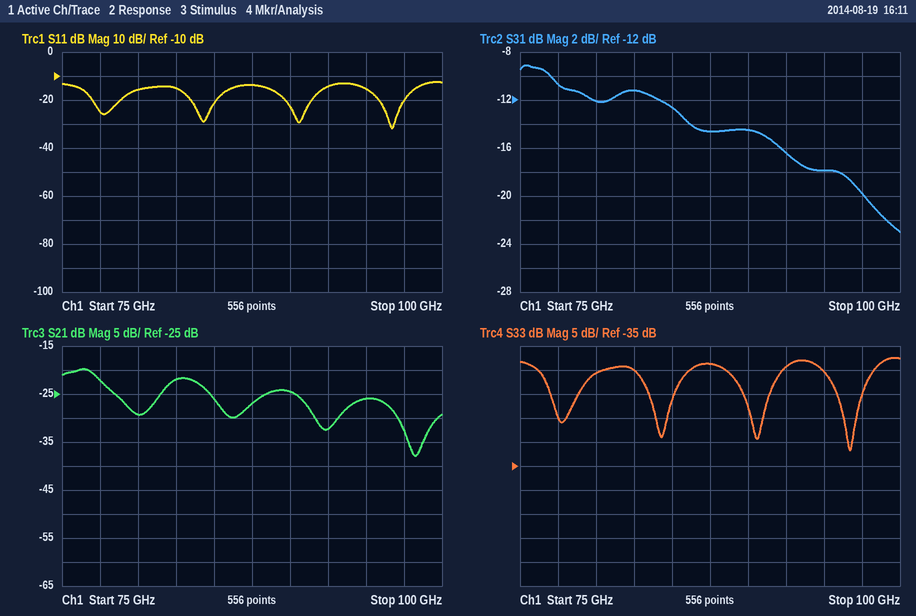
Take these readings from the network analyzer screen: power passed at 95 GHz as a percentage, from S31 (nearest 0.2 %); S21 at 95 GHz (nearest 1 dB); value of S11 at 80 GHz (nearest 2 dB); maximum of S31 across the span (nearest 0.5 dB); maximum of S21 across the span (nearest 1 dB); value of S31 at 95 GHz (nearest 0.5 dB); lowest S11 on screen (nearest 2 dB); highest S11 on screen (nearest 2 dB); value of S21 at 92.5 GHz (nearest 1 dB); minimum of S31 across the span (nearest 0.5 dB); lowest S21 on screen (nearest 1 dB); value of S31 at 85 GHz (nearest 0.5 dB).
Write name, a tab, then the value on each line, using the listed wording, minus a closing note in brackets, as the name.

power passed at 95 GHz as a percentage, from S31	1.6 %
S21 at 95 GHz	-26 dB
value of S11 at 80 GHz	-16 dB
maximum of S31 across the span	-9.0 dB
maximum of S21 across the span	-20 dB
value of S31 at 95 GHz	-18.0 dB
lowest S11 on screen	-32 dB
highest S11 on screen	-12 dB
value of S21 at 92.5 GHz	-32 dB
minimum of S31 across the span	-23.0 dB
lowest S21 on screen	-38 dB
value of S31 at 85 GHz	-12.5 dB
